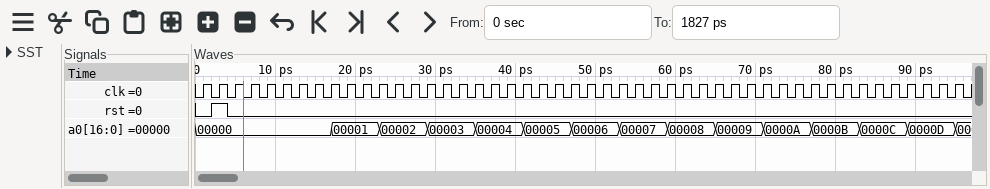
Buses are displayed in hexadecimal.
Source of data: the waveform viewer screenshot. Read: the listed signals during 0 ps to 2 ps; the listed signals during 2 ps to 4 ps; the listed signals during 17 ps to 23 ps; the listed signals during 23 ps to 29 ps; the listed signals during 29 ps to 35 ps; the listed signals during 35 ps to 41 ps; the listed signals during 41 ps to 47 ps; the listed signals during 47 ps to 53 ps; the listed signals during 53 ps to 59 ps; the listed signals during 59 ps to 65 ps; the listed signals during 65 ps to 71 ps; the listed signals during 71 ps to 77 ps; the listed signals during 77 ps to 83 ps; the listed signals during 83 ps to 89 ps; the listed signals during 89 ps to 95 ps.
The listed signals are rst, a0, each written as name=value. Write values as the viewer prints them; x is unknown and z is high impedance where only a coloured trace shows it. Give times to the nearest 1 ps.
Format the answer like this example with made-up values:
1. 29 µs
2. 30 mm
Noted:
1. rst=0, a0=00000
2. rst=1, a0=00000
3. rst=0, a0=00001
4. rst=0, a0=00002
5. rst=0, a0=00003
6. rst=0, a0=00004
7. rst=0, a0=00005
8. rst=0, a0=00006
9. rst=0, a0=00007
10. rst=0, a0=00008
11. rst=0, a0=00009
12. rst=0, a0=0000A
13. rst=0, a0=0000B
14. rst=0, a0=0000C
15. rst=0, a0=0000D
